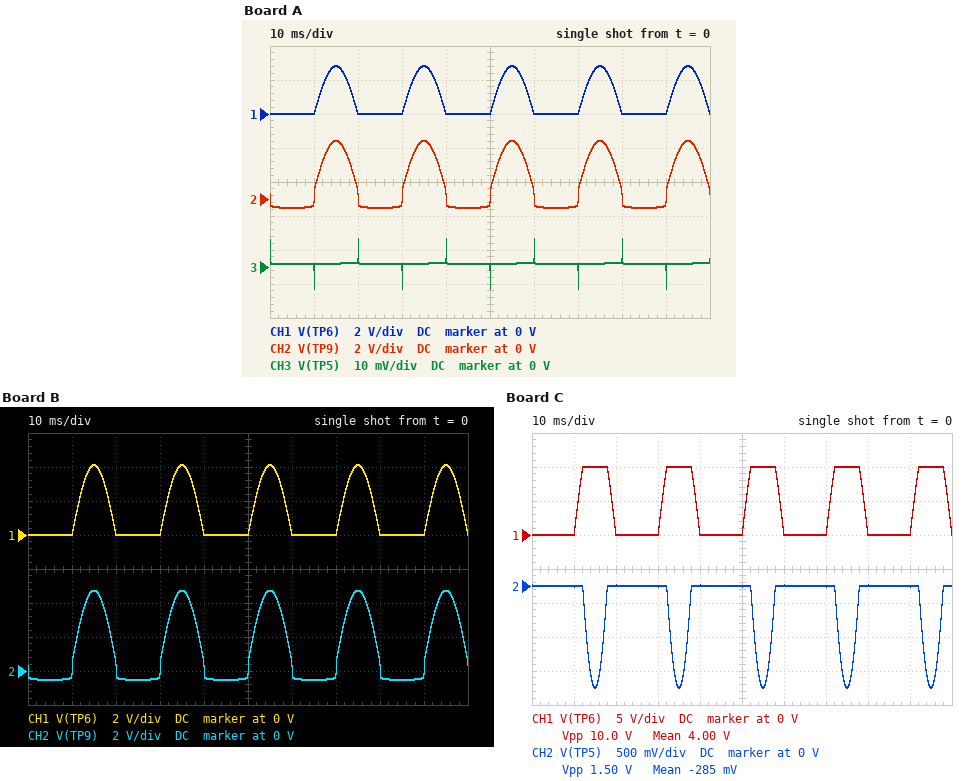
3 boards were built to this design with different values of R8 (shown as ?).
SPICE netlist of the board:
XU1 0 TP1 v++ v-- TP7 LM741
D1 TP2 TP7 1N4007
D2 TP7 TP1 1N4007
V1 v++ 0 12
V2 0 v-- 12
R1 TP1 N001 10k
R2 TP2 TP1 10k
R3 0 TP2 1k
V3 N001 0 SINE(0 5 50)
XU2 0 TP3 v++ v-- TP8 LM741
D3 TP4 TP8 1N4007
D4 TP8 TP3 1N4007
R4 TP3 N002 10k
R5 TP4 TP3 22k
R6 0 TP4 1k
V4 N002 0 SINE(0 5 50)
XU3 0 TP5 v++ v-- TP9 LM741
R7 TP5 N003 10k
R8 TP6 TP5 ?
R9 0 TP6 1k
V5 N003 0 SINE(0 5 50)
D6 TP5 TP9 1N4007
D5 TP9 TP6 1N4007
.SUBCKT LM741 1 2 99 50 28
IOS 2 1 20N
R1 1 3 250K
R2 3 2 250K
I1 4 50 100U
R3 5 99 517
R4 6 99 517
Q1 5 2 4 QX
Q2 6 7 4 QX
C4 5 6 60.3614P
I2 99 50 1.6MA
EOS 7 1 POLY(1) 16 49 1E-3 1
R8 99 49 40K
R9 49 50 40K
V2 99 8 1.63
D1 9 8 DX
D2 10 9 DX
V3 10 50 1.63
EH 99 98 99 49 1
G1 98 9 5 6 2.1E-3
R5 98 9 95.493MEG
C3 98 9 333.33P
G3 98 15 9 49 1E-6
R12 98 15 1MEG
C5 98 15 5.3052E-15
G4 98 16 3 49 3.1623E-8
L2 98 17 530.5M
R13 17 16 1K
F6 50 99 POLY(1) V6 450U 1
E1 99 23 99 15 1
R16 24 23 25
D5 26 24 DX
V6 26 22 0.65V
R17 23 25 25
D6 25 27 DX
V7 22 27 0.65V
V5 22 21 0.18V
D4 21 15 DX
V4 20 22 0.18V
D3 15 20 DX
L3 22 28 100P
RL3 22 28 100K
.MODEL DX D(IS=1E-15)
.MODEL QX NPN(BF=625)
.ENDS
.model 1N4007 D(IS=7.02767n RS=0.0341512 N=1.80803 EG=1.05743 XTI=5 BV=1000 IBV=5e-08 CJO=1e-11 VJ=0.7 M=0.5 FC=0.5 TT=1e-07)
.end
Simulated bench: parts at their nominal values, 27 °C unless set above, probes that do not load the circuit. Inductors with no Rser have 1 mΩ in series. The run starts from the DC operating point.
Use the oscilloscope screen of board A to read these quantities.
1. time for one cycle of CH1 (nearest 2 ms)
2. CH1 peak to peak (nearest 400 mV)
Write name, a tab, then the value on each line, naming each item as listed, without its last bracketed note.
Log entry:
time for one cycle of CH1	20 ms
CH1 peak to peak	2.8 V
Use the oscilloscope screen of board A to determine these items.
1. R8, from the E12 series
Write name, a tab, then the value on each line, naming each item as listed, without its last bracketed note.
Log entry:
R8, from the E12 series	5.6 kΩ
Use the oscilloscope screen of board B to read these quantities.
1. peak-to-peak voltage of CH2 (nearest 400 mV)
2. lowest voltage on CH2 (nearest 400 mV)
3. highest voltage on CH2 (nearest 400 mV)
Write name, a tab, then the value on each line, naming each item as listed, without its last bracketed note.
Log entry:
peak-to-peak voltage of CH2	5.2 V
lowest voltage on CH2	-400 mV
highest voltage on CH2	4.8 V
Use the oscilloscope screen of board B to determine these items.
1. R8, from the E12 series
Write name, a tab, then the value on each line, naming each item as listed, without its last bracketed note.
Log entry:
R8, from the E12 series	8.2 kΩ
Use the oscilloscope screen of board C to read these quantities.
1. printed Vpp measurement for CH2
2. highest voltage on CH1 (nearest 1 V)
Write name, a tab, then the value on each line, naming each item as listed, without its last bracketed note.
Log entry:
printed Vpp measurement for CH2	1.50 V
highest voltage on CH1	10 V
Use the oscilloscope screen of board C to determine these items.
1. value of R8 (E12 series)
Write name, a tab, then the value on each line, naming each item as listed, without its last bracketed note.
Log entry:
value of R8	33 kΩ
